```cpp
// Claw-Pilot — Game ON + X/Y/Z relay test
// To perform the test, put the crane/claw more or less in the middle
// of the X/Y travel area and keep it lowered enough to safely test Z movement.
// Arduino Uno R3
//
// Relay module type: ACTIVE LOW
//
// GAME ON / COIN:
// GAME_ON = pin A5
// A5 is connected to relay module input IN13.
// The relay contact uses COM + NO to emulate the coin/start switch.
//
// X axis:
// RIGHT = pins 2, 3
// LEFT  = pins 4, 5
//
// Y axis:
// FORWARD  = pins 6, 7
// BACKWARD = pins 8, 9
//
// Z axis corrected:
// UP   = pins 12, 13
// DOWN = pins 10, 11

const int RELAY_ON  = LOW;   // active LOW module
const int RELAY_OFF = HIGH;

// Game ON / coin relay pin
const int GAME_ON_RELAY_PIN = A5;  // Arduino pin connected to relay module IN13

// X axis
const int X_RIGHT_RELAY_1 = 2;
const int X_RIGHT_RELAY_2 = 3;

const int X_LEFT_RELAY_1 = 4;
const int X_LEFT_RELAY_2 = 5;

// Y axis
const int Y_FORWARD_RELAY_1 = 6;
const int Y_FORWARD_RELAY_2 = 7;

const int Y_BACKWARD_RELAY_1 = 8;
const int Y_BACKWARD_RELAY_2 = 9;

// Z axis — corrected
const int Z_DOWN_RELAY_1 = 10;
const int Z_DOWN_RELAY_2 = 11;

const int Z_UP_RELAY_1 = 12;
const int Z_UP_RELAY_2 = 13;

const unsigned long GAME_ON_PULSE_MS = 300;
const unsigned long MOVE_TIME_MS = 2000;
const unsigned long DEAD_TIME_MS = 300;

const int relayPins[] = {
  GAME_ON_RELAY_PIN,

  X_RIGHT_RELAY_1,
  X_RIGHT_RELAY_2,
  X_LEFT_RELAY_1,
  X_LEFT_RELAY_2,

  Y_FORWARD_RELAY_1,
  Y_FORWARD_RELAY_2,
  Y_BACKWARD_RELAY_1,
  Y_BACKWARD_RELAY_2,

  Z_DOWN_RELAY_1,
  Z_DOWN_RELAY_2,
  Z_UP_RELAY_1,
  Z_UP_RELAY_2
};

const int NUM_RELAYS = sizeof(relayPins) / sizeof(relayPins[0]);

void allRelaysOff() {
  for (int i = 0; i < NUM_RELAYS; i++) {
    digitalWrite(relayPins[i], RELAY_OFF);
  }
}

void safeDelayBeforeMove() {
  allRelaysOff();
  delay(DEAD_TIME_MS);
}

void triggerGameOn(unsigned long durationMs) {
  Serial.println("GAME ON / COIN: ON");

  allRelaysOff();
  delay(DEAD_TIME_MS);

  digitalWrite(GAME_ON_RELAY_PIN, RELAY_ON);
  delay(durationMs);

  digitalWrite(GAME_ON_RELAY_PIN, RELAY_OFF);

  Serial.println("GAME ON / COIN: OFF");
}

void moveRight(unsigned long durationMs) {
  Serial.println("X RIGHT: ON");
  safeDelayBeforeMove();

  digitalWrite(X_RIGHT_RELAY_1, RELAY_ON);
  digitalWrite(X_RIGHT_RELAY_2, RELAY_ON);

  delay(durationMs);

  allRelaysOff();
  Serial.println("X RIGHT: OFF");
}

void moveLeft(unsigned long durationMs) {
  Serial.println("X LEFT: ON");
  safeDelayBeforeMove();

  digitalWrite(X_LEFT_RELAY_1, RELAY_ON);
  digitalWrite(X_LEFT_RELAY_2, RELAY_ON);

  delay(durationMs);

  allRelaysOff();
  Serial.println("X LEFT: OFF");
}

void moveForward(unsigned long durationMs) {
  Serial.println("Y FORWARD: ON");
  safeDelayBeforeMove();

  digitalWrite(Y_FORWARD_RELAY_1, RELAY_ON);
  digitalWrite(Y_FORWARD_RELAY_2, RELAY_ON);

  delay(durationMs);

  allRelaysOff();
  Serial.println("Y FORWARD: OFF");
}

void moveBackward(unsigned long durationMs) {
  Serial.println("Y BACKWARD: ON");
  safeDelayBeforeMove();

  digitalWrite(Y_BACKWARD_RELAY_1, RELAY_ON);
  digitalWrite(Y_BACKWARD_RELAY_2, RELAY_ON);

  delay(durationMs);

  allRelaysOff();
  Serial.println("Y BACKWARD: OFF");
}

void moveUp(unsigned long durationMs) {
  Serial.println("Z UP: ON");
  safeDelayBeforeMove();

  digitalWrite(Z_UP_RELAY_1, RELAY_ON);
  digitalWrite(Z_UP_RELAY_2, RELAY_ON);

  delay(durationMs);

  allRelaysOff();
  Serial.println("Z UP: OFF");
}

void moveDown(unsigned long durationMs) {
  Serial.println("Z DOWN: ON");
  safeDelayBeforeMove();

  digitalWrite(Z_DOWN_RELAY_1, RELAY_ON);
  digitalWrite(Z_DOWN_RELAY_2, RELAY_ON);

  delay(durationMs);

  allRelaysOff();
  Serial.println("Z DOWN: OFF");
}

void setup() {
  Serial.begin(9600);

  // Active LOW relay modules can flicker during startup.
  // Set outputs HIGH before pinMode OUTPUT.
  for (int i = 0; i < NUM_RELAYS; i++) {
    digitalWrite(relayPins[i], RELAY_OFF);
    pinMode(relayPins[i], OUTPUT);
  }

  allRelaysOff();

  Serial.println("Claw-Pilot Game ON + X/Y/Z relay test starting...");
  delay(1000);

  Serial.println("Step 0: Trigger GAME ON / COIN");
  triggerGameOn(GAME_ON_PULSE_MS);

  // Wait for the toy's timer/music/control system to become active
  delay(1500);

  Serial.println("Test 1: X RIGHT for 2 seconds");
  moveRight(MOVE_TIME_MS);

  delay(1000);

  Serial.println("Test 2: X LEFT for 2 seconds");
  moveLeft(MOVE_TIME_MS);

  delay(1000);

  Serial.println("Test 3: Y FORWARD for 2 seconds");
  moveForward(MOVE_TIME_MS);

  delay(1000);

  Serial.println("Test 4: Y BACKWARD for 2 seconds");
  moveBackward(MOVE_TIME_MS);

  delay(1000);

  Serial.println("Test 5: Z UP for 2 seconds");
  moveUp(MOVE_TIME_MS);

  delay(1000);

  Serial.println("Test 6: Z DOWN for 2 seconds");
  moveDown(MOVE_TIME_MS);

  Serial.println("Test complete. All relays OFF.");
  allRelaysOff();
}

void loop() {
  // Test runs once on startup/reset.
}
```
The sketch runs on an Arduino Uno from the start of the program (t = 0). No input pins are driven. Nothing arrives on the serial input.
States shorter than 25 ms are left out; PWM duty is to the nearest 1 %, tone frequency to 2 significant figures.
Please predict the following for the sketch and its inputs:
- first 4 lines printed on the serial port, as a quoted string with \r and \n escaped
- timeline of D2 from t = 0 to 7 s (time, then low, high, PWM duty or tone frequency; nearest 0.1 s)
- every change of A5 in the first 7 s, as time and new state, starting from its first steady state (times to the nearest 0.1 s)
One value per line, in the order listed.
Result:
"Claw-Pilot Game ON + X/Y/Z relay test starting...\r\nStep 0: Trigger GAME ON / COIN\r\nGAME ON / COIN: ON\r\nGAME ON / COIN: OFF\r\n"
0 s high; 3.4 s low; 5.4 s high
0 s high; 1.3 s low; 1.6 s high
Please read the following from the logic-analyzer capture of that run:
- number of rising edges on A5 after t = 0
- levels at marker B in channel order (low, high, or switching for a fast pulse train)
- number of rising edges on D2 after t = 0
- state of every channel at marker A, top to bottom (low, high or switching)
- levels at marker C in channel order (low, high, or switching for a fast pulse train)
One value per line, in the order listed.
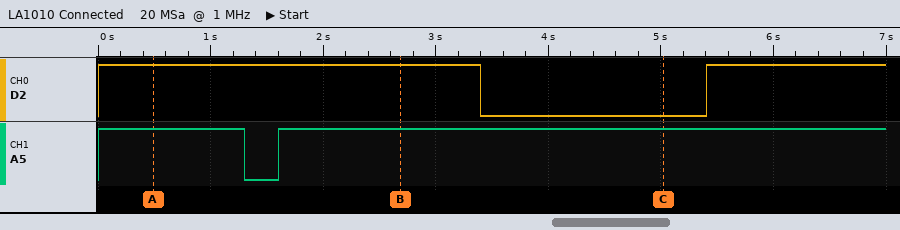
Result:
1
D2 high, A5 high
1
D2 high, A5 high
D2 low, A5 high
